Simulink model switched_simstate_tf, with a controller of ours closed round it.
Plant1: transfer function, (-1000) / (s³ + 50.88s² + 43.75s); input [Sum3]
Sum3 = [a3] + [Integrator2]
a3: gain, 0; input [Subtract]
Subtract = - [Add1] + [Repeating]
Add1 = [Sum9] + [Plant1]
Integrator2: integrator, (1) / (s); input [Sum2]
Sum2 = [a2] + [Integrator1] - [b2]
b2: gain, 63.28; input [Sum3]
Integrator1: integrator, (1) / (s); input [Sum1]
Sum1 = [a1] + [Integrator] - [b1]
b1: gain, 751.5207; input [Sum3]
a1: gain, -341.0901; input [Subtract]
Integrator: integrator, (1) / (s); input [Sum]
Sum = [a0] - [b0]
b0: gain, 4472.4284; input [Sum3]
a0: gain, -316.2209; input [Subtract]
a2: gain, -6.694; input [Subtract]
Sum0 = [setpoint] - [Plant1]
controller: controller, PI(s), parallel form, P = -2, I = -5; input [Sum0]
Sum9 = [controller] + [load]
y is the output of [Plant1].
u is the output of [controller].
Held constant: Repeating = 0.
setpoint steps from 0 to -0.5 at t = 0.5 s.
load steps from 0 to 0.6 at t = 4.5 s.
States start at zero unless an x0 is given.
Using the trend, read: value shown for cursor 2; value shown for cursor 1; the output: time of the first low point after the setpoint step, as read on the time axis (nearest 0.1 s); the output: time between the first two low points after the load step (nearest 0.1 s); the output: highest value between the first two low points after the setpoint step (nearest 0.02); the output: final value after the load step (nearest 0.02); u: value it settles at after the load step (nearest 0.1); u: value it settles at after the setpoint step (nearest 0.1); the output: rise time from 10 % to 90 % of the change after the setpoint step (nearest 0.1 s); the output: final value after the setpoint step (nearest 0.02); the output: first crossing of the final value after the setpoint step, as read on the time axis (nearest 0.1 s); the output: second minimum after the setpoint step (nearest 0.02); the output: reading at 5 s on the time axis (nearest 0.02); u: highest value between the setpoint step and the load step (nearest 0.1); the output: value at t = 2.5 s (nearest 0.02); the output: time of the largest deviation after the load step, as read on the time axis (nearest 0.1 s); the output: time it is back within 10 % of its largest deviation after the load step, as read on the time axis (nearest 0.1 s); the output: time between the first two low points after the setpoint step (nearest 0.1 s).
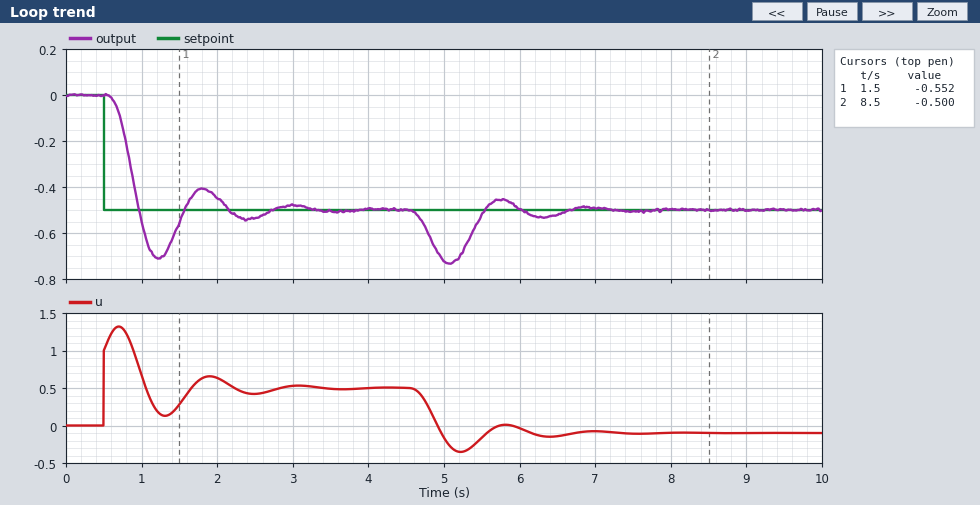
-0.500
-0.552
1.2 s
1.2 s
-0.40
-0.50
-0.1
0.5
0.3 s
-0.50
1.0 s
-0.54
-0.72
1.3
-0.54
5.1 s
6.5 s
1.2 s
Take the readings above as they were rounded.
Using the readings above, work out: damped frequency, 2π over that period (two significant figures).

5.2 rad/s
